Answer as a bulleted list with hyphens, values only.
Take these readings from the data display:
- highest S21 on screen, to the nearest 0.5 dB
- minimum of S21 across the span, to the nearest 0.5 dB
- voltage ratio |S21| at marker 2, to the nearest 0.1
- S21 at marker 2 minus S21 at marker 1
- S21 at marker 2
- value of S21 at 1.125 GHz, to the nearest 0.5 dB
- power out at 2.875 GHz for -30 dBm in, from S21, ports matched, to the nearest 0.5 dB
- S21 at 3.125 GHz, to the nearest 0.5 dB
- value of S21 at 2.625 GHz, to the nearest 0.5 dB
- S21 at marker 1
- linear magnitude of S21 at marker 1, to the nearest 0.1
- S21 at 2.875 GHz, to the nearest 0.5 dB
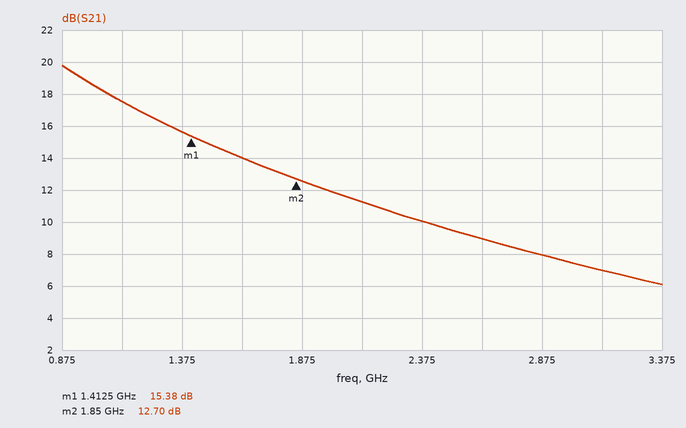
- 20.0 dB
- 6.0 dB
- 4.3
- -2.68 dB
- 12.70 dB
- 17.5 dB
- -22.0 dBm
- 7.0 dB
- 9.0 dB
- 15.38 dB
- 5.9
- 8.0 dB
